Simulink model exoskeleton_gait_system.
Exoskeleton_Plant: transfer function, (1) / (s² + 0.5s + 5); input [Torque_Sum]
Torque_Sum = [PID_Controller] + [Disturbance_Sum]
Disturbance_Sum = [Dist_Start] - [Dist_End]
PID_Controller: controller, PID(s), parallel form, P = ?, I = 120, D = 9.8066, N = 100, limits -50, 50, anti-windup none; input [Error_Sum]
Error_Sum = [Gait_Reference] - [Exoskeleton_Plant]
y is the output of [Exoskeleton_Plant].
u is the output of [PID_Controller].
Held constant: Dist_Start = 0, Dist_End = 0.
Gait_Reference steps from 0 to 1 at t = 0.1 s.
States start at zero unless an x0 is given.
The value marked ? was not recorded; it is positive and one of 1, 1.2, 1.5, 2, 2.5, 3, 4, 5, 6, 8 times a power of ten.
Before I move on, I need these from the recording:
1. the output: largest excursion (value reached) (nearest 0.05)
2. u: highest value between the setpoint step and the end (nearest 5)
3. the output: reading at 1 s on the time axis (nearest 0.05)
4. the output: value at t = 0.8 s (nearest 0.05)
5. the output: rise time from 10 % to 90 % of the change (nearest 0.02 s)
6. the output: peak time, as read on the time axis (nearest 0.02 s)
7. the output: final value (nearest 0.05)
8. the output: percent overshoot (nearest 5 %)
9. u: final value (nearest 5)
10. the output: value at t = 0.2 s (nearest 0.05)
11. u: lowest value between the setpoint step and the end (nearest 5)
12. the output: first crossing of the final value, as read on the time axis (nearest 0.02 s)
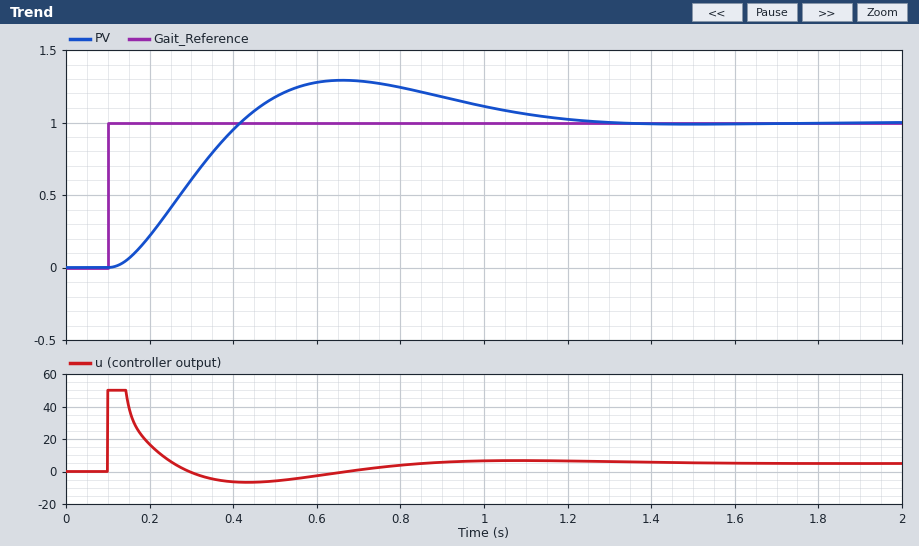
1.30
50
1.10
1.25
0.22 s
0.66 s
1.00
30 %
5
0.20
-5
0.42 s
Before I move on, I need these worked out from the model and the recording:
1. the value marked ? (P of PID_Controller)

50
